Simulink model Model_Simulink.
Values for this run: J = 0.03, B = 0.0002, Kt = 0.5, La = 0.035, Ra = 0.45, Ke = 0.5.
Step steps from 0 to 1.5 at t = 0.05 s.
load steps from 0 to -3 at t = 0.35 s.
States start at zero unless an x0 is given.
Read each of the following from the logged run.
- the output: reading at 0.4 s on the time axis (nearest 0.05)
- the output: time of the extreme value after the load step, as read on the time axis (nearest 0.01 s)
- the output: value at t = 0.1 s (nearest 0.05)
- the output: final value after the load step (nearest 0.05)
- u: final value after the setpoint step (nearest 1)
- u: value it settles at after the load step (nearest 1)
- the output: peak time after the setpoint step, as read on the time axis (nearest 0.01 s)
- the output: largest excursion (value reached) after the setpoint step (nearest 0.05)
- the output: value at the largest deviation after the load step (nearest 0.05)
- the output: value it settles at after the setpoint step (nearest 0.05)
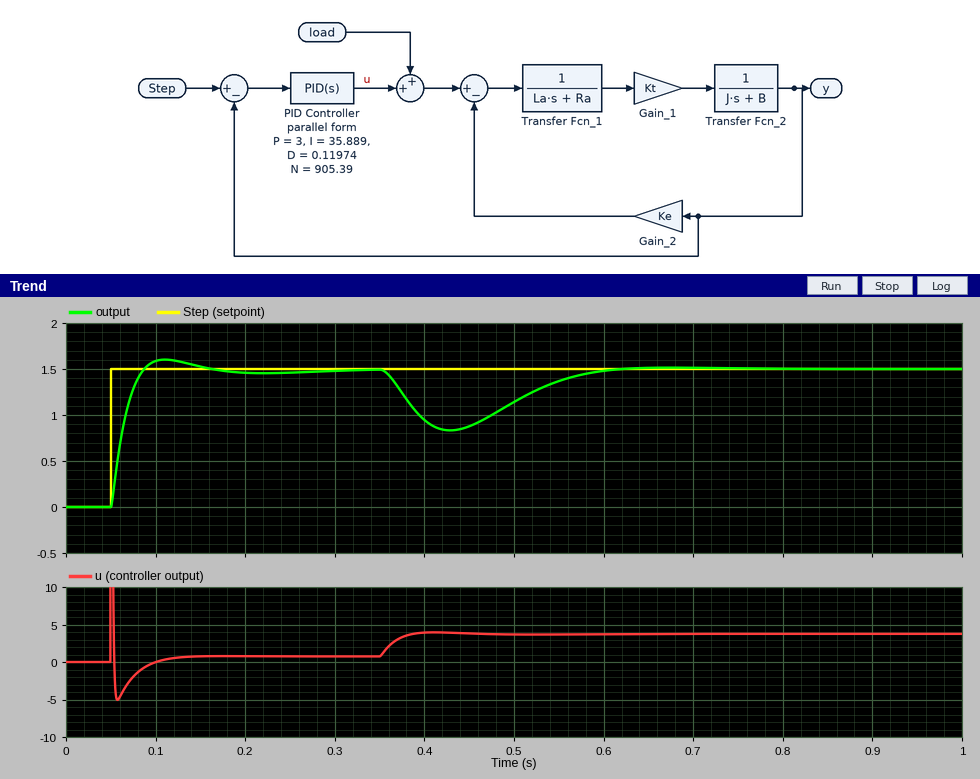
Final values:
0.95
0.43 s
1.60
1.50
1
4
0.11 s
1.60
0.85
1.50
